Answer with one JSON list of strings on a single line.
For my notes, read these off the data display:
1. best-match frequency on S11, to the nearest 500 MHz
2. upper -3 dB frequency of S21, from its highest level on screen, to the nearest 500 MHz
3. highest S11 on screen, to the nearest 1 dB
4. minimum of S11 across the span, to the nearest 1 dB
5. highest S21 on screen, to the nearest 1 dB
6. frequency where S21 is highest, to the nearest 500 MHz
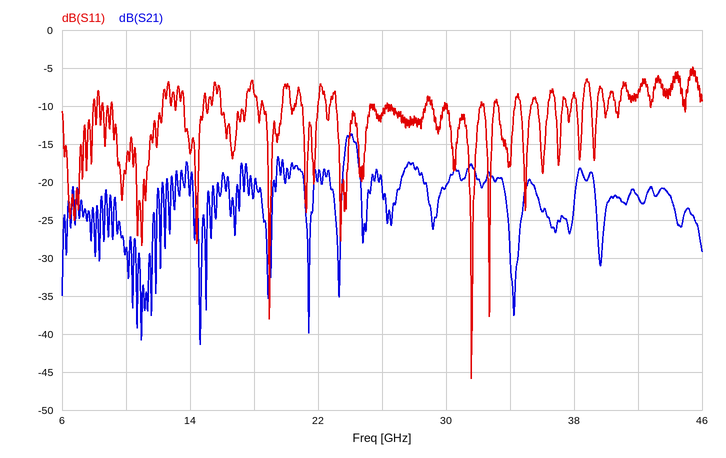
["31.5 GHz", "24.5 GHz", "-5 dB", "-46 dB", "-14 dB", "24.0 GHz"]
